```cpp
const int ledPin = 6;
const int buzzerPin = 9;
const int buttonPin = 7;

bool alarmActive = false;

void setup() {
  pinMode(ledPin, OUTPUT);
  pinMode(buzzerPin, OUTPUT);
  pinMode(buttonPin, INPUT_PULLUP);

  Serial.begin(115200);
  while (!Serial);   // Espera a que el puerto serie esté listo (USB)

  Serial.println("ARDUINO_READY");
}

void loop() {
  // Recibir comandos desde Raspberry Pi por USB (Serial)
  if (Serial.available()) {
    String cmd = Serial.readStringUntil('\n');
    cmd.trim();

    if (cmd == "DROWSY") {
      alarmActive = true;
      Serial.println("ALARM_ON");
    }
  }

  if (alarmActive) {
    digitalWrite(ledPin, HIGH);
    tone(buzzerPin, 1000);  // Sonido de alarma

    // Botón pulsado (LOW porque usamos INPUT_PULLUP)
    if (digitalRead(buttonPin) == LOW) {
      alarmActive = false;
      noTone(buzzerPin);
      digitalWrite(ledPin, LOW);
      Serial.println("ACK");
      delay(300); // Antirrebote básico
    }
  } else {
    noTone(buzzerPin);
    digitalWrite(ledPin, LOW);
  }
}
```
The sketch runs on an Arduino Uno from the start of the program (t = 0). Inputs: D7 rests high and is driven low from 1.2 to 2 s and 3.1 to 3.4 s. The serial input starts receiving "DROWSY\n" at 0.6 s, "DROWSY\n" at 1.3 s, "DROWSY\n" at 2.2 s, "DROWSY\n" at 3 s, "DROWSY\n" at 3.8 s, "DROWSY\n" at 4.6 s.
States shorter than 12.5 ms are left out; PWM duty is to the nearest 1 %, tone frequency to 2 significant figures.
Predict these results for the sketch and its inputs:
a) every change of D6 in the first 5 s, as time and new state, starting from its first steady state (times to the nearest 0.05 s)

0 s low; 0.6 s high; 1.2 s low; 2.2 s high; 3.1 s low; 3.8 s high
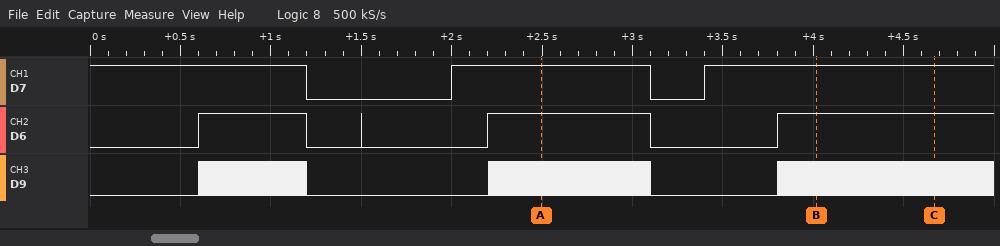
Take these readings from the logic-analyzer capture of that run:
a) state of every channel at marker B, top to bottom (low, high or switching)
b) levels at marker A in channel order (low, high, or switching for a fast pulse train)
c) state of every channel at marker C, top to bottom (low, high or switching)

D7 high, D6 high, D9 switching
D7 high, D6 high, D9 switching
D7 high, D6 high, D9 switching
